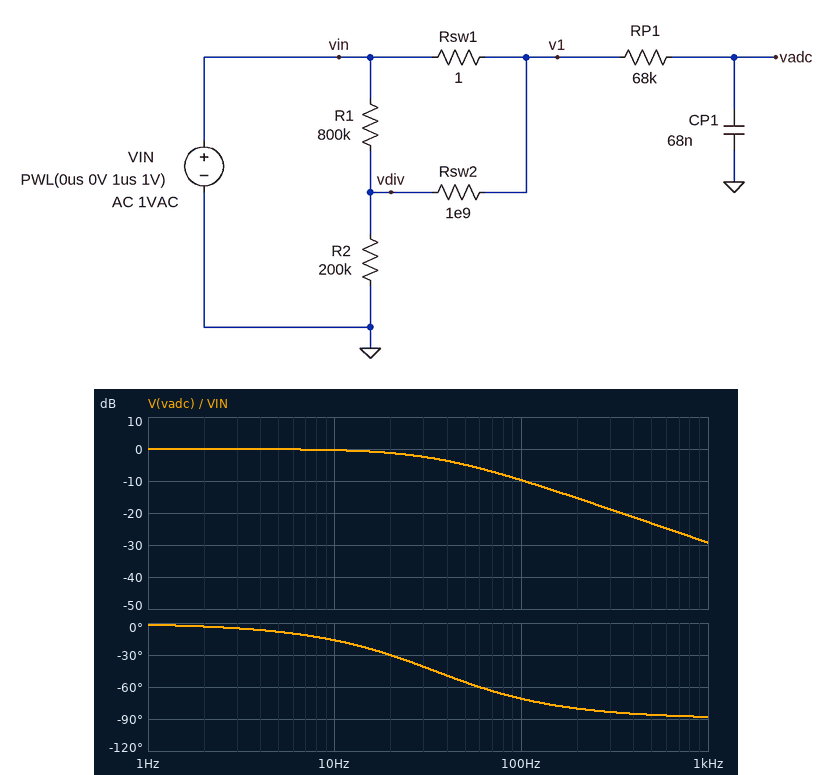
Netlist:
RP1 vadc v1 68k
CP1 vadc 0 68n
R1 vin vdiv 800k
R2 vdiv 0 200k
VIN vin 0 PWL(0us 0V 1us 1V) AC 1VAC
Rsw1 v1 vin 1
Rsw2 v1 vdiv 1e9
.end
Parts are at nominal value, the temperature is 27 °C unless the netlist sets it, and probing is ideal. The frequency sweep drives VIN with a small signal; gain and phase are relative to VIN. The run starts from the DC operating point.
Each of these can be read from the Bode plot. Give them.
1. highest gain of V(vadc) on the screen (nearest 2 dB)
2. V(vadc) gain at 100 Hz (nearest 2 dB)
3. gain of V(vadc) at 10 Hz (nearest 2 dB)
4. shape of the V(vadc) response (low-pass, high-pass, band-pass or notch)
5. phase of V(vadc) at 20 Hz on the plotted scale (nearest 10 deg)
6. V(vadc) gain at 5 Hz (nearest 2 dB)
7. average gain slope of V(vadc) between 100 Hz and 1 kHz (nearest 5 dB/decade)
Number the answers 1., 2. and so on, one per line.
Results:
1. 0 dB
2. -10 dB
3. 0 dB
4. low-pass
5. -30 deg
6. 0 dB
7. -20 dB/decade
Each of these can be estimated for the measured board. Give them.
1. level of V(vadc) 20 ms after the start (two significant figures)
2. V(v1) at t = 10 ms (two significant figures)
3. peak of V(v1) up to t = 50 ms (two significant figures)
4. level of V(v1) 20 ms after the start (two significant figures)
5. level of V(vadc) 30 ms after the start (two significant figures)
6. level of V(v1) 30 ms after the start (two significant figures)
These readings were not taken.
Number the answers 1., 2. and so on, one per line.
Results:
1. 990 mV
2. 1.0 V
3. 1.0 V
4. 1.0 V
5. 1.0 V
6. 1.0 V
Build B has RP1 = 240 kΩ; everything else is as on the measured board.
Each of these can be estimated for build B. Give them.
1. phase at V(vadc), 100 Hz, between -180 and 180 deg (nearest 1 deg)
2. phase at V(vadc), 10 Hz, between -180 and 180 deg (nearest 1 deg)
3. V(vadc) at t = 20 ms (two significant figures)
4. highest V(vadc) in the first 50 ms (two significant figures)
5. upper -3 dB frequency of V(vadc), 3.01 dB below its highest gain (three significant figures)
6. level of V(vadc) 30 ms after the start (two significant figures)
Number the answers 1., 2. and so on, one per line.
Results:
1. -84 deg
2. -46 deg
3. 710 mV
4. 950 mV
5. 9.75 Hz
6. 840 mV
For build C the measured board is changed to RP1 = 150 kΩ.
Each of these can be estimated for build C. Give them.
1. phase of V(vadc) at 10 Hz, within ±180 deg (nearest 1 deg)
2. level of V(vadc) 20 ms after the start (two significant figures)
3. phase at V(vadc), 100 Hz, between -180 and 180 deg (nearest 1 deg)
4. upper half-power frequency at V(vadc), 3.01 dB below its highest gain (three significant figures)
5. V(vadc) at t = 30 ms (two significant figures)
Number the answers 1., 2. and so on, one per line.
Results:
1. -33 deg
2. 860 mV
3. -81 deg
4. 15.6 Hz
5. 950 mV
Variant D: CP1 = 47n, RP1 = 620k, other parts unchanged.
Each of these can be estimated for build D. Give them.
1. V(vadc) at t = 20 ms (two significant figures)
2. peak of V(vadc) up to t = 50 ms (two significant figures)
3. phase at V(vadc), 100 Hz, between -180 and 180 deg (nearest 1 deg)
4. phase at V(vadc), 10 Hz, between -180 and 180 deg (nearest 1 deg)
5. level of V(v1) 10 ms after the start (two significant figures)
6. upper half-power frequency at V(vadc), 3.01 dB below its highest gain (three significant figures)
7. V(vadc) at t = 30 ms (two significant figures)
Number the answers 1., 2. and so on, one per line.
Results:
1. 500 mV
2. 820 mV
3. -87 deg
4. -61 deg
5. 1.0 V
6. 5.46 Hz
7. 640 mV
